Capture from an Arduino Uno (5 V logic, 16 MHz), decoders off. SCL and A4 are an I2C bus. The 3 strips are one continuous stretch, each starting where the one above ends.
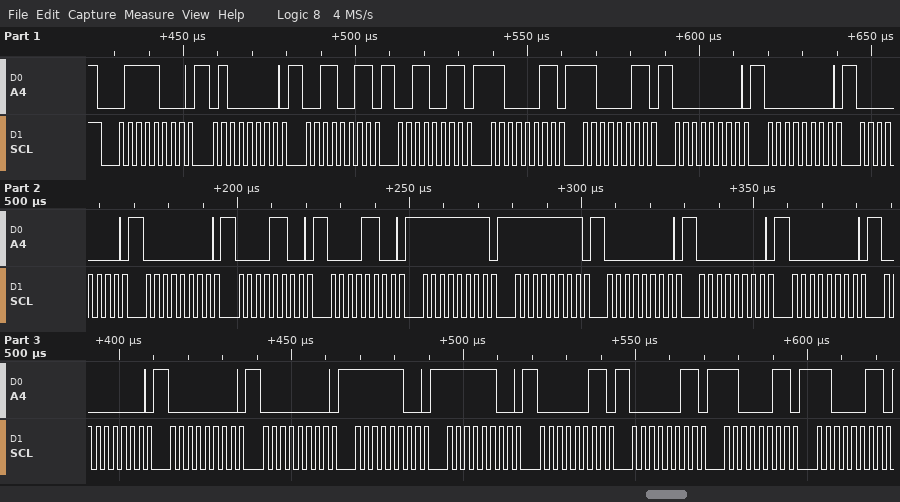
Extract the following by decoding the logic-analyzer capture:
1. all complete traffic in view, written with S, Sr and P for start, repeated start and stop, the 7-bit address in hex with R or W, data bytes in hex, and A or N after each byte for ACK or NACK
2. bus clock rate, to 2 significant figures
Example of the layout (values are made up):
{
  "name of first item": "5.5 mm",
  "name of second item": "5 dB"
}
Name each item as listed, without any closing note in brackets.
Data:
{
  "all complete traffic in view, written with S, Sr and P for start, repeated start and stop, the 7-bit address in hex with R or W, data bytes in hex, and A or N after each byte for ACK or NACK": "S 3CW A 40 A 33 A 33 A C3 A C3 A 00 A 00 A 00 A 00 A 0C A 0C A FF A FF A 00 A 00 A 00 A 00 A 00 A 00 A FC A FC A 03 A 03 A C3 A C3 A",
  "bus clock rate, to 2 significant figures": "400 kHz"
}
